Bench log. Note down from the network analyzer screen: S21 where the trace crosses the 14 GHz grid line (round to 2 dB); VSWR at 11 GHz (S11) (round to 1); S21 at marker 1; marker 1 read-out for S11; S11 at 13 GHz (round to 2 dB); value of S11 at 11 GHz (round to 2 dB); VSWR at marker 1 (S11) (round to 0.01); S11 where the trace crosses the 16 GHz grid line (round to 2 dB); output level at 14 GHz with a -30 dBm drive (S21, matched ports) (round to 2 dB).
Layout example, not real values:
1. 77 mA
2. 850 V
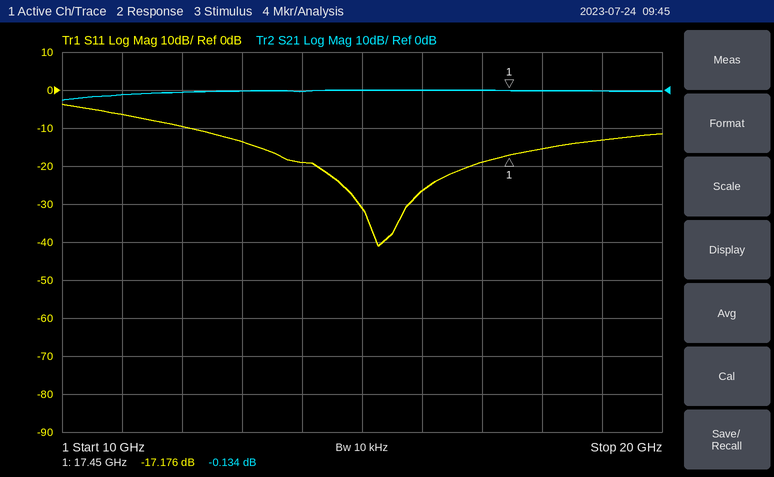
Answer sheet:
1. 0 dB
2. 3
3. -0.134 dB
4. -17.176 dB
5. -14 dB
6. -6 dB
7. 1.32
8. -26 dB
9. -30 dBm
